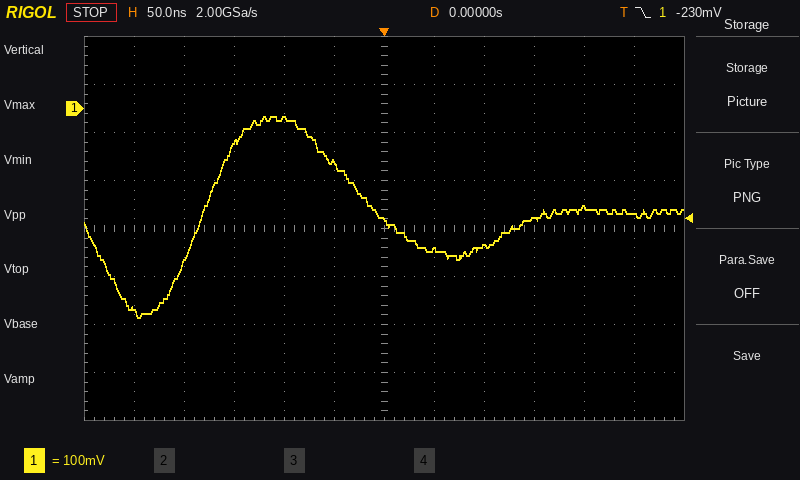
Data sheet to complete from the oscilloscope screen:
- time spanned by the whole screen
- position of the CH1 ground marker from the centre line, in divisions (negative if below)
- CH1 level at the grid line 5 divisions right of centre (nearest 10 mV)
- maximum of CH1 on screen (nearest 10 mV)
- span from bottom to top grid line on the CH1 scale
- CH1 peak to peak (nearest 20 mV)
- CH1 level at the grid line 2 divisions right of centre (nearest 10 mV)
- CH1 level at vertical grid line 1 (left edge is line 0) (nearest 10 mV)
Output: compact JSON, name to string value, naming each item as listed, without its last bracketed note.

{"time spanned by the whole screen": "600 ns", "position of the CH1 ground marker from the centre line, in divisions": "+2.5 div", "CH1 level at the grid line 5 divisions right of centre": "-220 mV", "maximum of CH1 on screen": "-20 mV", "span from bottom to top grid line on the CH1 scale": "800 mV", "CH1 peak to peak": "420 mV", "CH1 level at the grid line 2 divisions right of centre": "-290 mV", "CH1 level at vertical grid line 1 (left edge is line 0)": "-420 mV"}
